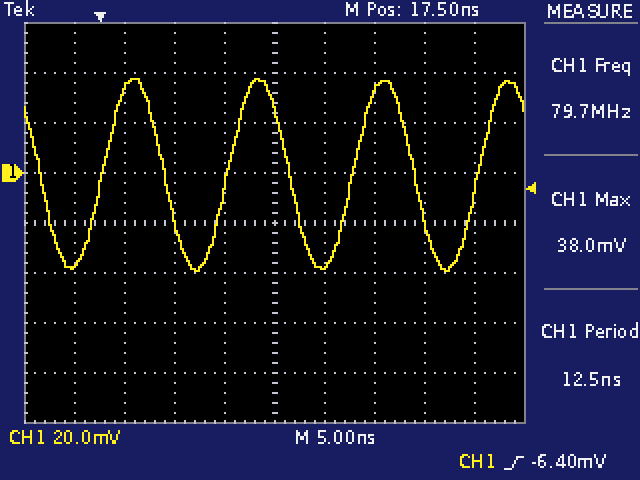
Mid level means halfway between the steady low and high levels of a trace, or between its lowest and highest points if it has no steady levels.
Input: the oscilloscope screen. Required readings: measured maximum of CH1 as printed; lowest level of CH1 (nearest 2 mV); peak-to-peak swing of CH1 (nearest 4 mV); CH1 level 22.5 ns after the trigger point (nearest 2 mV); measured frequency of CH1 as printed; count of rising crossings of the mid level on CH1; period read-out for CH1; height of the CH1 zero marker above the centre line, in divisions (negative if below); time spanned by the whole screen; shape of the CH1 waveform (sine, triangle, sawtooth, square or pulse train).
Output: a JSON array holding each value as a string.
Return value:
["38.0 mV", "-40 mV", "76 mV", "-38 mV", "79.7 MHz", "4", "12.5 ns", "+1.0 div", "50 ns", "sine"]
